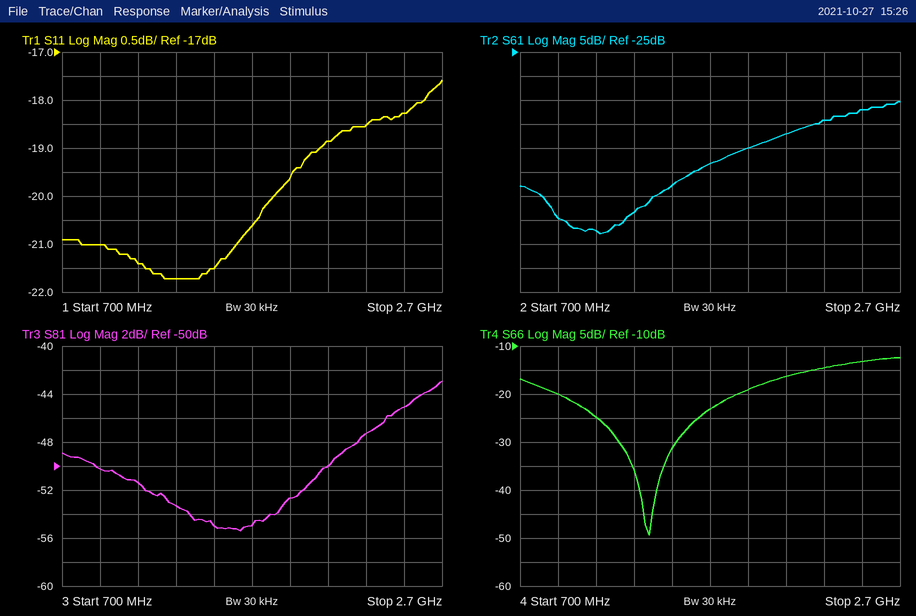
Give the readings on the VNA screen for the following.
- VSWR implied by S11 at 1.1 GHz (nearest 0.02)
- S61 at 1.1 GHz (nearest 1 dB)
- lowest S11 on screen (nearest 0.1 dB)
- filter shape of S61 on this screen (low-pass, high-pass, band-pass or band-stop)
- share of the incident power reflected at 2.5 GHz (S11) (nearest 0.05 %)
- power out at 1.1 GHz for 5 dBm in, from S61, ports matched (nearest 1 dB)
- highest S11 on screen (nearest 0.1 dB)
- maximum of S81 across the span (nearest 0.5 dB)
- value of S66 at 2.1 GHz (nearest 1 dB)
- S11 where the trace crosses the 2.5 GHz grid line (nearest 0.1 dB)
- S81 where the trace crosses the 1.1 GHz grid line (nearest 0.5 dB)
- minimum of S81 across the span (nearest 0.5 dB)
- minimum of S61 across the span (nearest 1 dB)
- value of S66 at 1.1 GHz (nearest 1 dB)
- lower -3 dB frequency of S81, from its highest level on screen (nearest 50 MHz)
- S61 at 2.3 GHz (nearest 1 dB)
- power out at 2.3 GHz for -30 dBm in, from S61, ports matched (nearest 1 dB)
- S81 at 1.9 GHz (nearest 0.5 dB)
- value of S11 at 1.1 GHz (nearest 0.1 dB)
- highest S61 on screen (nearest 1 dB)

1.18
-62 dB
-21.7 dB
high-pass
1.50 %
-57 dBm
-17.6 dB
-43.0 dB
-16 dB
-18.3 dB
-51.5 dB
-55.5 dB
-63 dB
-25 dB
2.40 GHz
-39 dB
-69 dBm
-52.5 dB
-21.4 dB
-35 dB
